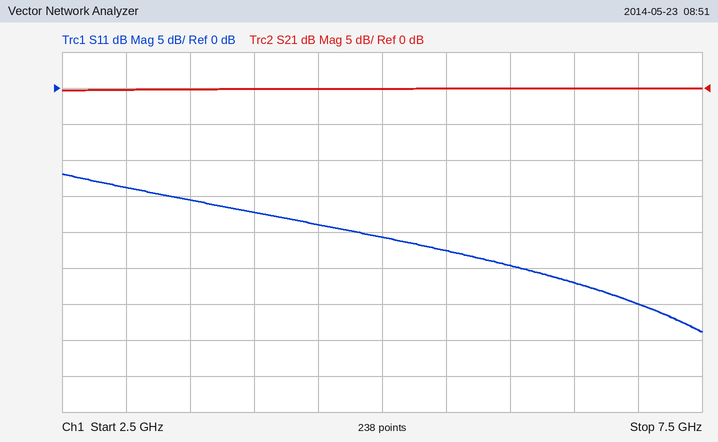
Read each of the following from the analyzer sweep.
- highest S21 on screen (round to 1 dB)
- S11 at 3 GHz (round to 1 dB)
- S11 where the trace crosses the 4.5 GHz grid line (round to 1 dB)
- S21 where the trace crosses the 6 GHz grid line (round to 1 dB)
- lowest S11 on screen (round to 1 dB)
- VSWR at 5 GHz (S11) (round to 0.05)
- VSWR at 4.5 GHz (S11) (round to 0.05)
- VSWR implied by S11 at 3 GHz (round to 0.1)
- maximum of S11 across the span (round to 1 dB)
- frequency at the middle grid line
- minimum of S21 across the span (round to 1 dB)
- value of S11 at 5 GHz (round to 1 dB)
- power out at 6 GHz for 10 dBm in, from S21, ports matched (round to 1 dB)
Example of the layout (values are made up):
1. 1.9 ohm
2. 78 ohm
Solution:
1. 0 dB
2. -14 dB
3. -19 dB
4. 0 dB
5. -34 dB
6. 1.20
7. 1.25
8. 1.5
9. -12 dB
10. 5 GHz
11. 0 dB
12. -21 dB
13. 10 dBm
